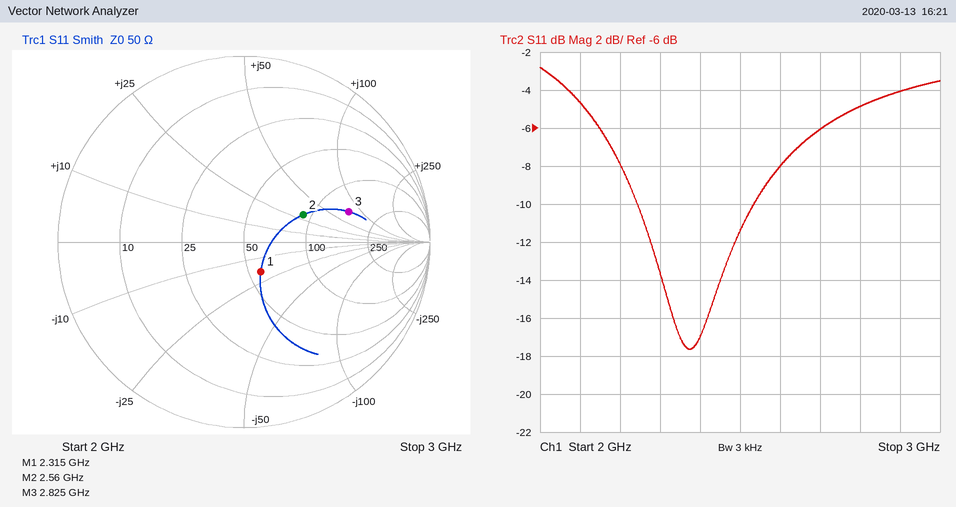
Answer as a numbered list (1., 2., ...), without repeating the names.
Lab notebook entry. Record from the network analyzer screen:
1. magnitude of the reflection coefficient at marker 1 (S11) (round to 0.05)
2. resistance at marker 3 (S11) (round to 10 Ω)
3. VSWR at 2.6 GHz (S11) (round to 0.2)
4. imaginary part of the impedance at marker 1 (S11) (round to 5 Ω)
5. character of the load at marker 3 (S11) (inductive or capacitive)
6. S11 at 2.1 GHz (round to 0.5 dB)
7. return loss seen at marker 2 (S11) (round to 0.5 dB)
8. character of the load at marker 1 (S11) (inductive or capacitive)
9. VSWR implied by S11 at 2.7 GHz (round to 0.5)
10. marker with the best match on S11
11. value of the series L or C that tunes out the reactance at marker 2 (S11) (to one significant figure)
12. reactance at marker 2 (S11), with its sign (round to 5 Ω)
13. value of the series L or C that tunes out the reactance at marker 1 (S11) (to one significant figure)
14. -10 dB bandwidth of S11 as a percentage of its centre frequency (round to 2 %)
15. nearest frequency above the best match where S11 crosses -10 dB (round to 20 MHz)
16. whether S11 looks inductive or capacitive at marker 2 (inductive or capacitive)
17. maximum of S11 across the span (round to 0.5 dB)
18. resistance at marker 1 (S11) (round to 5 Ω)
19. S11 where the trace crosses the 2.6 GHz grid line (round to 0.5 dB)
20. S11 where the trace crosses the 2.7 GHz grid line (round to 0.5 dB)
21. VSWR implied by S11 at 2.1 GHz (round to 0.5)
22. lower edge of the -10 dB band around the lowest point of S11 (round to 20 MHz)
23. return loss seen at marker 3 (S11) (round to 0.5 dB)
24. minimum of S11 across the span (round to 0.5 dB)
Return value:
1. 0.20
2. 150 Ω
3. 2.4
4. -20 Ω
5. inductive
6. -4.5 dB
7. 9.0 dB
8. capacitive
9. 3.0
10. marker 1
11. 2 pF
12. +30 Ω
13. 1 nH
14. 12 %
15. 2.54 GHz
16. inductive
17. -3.0 dB
18. 55 Ω
19. -8.0 dB
20. -6.0 dB
21. 4.0
22. 2.24 GHz
23. 4.5 dB
24. -17.5 dB
